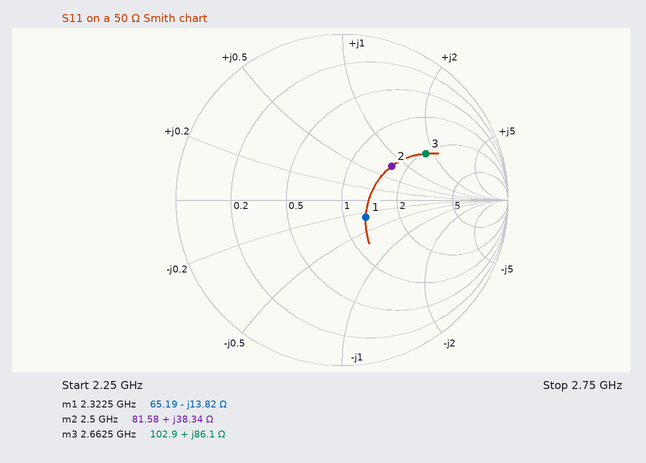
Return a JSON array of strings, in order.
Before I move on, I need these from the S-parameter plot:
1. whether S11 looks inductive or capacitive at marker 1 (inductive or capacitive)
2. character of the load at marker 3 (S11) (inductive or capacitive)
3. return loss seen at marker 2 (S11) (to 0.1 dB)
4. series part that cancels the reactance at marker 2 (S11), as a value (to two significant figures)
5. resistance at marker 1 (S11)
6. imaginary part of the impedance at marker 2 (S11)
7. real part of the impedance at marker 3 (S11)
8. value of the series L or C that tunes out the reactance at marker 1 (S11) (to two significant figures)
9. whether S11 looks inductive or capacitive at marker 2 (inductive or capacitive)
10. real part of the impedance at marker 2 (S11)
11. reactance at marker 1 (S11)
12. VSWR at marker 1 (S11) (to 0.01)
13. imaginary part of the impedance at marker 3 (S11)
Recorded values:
["capacitive", "inductive", "8.8 dB", "1.7 pF", "65.19 Ω", "+38.34 Ω", "102.9 Ω", "950 pH", "inductive", "81.58 Ω", "-13.82 Ω", "1.43", "+86.1 Ω"]
